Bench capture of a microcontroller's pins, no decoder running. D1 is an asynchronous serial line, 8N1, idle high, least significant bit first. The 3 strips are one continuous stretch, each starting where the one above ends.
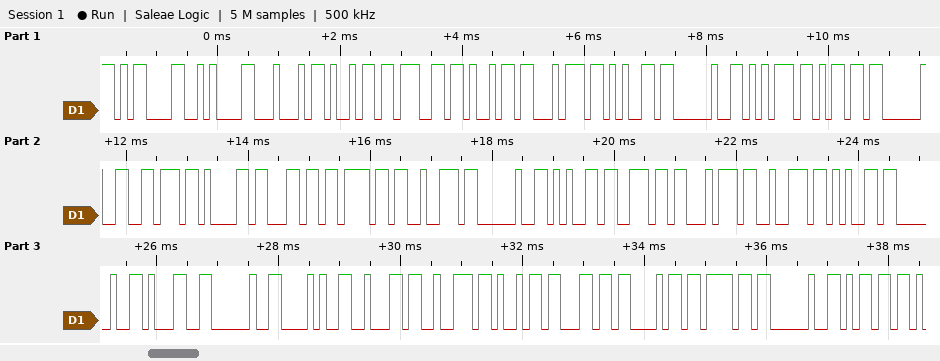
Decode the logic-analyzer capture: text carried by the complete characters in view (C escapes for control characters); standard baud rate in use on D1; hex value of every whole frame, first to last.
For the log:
"\r\nDigite um valor entre 1 (brilho m"
9600 baud
0x0D 0x0A 0x44 0x69 0x67 0x69 0x74 0x65 0x20 0x75 0x6D 0x20 0x76 0x61 0x6C 0x6F 0x72 0x20 0x65 0x6E 0x74 0x72 0x65 0x20 0x31 0x20 0x28 0x62 0x72 0x69 0x6C 0x68 0x6F 0x20 0x6D
